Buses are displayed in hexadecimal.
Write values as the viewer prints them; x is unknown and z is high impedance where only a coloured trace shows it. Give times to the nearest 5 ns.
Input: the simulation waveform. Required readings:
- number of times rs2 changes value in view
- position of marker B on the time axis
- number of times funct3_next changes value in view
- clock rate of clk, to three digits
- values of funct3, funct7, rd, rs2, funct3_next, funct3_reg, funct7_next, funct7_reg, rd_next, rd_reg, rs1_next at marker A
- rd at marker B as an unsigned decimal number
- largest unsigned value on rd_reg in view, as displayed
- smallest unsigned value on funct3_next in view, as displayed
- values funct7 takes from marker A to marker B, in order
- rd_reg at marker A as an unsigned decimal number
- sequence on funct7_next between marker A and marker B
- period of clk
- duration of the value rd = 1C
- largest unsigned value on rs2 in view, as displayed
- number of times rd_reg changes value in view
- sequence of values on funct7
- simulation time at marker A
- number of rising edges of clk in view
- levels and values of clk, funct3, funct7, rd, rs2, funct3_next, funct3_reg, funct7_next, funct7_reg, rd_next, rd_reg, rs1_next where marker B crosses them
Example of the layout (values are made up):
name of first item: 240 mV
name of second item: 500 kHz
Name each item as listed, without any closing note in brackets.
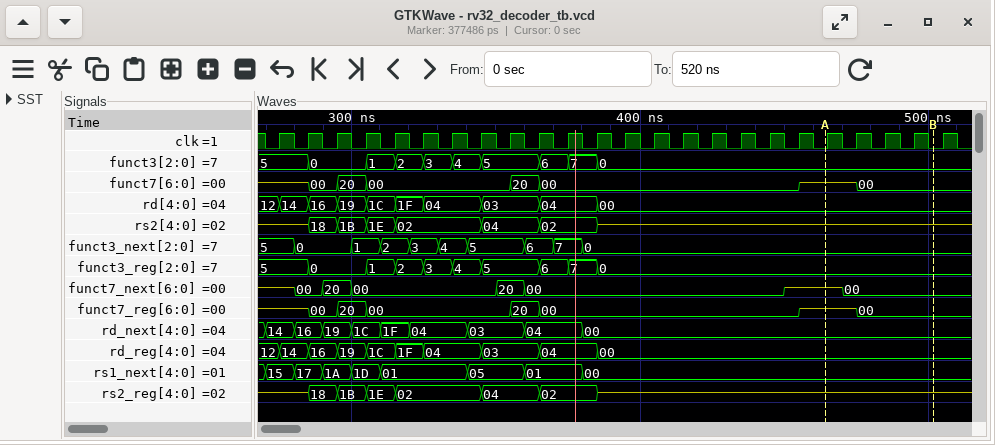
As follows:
number of times rs2 changes value in view: 7
position of marker B on the time axis: 500 ns
number of times funct3_next changes value in view: 9
clock rate of clk, to three digits: 100 MHz
values of funct3, funct7, rd, rs2, funct3_next, funct3_reg, funct7_next, funct7_reg, rd_next, rd_reg, rs1_next at marker A: funct3=0, funct7=z, rd=00, rs2=z, funct3_next=0, funct3_reg=0, funct7_next=z, funct7_reg=z, rd_next=00, rd_reg=00, rs1_next=00
rd at marker B as an unsigned decimal number: 0
largest unsigned value on rd_reg in view, as displayed: 1F
smallest unsigned value on funct3_next in view, as displayed: 0
values funct7 takes from marker A to marker B, in order: z, 00
rd_reg at marker A as an unsigned decimal number: 0
sequence on funct7_next between marker A and marker B: z, 00
period of clk: 10 ns
duration of the value rd = 1C: 10 ns
largest unsigned value on rs2 in view, as displayed: 1E
number of times rd_reg changes value in view: 9
sequence of values on funct7: z, 00, 20, 00, 20, 00, z, 00
simulation time at marker A: 465 ns
number of rising edges of clk in view: 24
levels and values of clk, funct3, funct7, rd, rs2, funct3_next, funct3_reg, funct7_next, funct7_reg, rd_next, rd_reg, rs1_next where marker B crosses them: clk=0, funct3=0, funct7=00, rd=00, rs2=z, funct3_next=0, funct3_reg=0, funct7_next=00, funct7_reg=00, rd_next=00, rd_reg=00, rs1_next=00
